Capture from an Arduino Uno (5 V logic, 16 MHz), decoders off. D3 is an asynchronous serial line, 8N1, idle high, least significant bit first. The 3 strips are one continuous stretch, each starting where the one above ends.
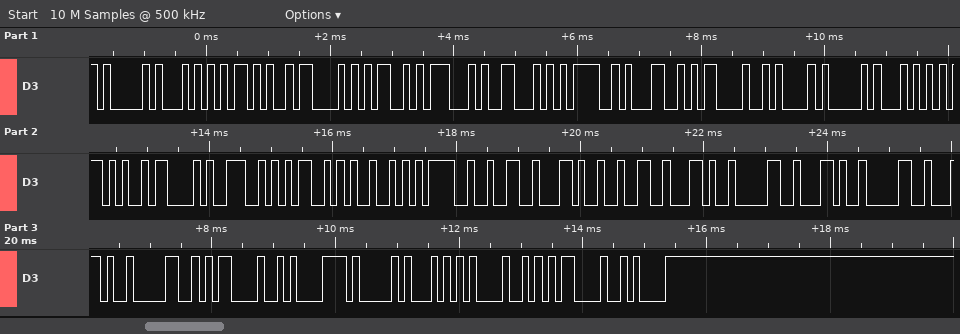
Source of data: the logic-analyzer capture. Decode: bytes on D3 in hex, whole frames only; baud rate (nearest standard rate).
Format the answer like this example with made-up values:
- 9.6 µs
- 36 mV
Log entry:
- 41 54 2B 43 4D 47 46 3D 31 0D 0A 41 54 2B 43 4E 4D 49 3D 32 2C 32 2C 30 2C 30 2C 30 0D 0A 41 54 48 0D 0A
- 9600 baud
